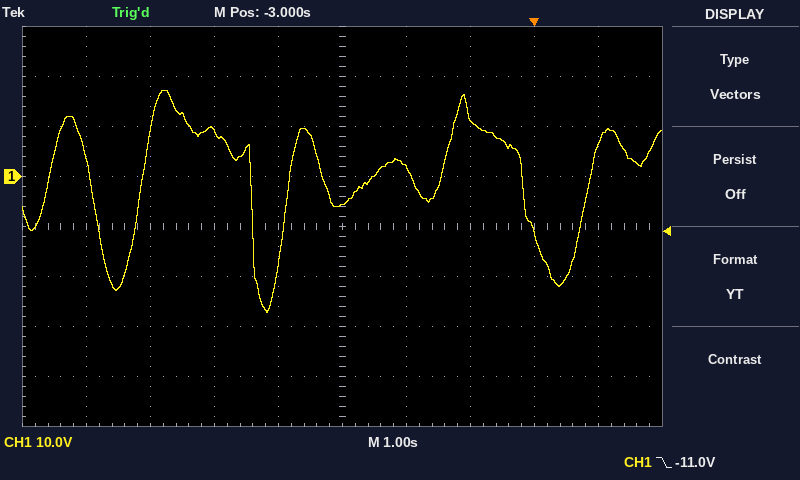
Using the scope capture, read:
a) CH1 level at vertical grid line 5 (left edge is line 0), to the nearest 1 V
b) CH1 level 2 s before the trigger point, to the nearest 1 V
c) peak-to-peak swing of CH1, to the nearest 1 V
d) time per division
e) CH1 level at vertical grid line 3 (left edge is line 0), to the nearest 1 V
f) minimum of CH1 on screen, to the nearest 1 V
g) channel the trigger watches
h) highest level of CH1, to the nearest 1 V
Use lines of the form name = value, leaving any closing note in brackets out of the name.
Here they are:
CH1 level at vertical grid line 5 (left edge is line 0), to the nearest 1 V = -6 V
CH1 level 2 s before the trigger point, to the nearest 1 V = 2 V
peak-to-peak swing of CH1, to the nearest 1 V = 44 V
time per division = 1 s
CH1 level at vertical grid line 3 (left edge is line 0), to the nearest 1 V = 9 V
minimum of CH1 on screen, to the nearest 1 V = -27 V
channel the trigger watches = CH1
highest level of CH1, to the nearest 1 V = 17 V
